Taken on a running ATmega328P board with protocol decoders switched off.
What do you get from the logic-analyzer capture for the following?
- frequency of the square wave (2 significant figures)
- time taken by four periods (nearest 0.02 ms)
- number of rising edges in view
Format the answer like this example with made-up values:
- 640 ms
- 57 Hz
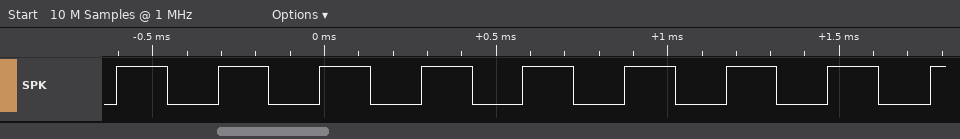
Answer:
- 3.4 kHz
- 1.18 ms
- 9
